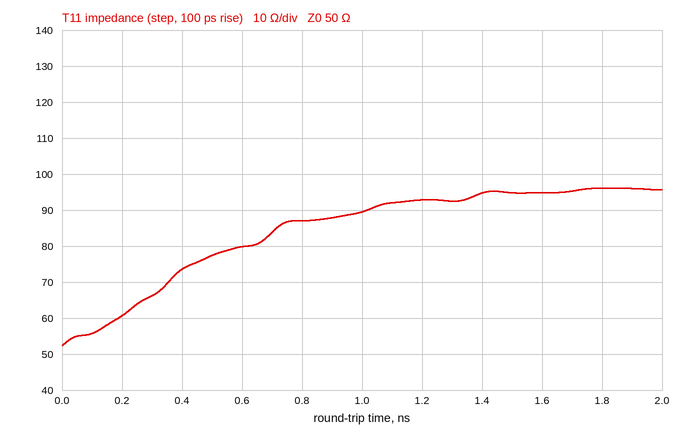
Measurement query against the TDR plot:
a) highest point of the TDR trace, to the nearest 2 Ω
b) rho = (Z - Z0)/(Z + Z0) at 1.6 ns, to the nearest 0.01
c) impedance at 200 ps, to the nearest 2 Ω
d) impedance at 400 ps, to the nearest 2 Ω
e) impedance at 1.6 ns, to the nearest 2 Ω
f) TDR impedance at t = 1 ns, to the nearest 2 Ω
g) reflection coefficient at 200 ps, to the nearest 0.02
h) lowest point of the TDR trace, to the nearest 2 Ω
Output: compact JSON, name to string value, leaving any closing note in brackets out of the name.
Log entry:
{"highest point of the TDR trace, to the nearest 2 Ω": "96 Ω", "rho = (Z - Z0)/(Z + Z0) at 1.6 ns, to the nearest 0.01": "+0.31", "impedance at 200 ps, to the nearest 2 Ω": "60 Ω", "impedance at 400 ps, to the nearest 2 Ω": "74 Ω", "impedance at 1.6 ns, to the nearest 2 Ω": "94 Ω", "TDR impedance at t = 1 ns, to the nearest 2 Ω": "90 Ω", "reflection coefficient at 200 ps, to the nearest 0.02": "+0.10", "lowest point of the TDR trace, to the nearest 2 Ω": "52 Ω"}
